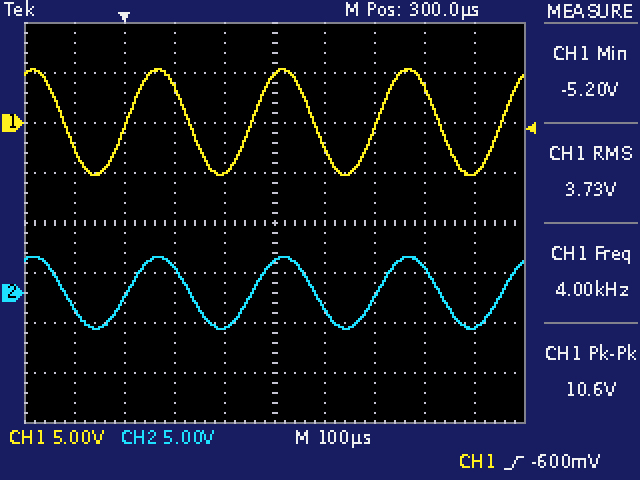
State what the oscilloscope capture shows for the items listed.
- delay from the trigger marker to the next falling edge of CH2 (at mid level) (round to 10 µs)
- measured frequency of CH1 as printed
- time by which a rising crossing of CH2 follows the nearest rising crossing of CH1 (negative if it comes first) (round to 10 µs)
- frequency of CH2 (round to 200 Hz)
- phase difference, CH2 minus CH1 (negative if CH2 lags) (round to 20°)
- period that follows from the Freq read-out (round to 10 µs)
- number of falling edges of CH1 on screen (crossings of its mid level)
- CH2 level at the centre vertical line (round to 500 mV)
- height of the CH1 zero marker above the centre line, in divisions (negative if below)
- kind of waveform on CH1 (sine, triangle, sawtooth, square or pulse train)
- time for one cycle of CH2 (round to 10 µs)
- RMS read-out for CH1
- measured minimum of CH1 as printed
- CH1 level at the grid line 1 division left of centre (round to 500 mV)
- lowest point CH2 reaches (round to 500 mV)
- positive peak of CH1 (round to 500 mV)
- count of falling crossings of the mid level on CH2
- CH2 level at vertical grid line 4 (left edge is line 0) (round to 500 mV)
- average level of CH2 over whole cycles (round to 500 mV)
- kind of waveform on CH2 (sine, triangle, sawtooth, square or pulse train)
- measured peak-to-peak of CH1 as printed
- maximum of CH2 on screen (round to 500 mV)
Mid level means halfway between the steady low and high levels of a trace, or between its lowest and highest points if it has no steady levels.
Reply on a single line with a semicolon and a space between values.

130 µs; 4.00 kHz; 0 µs; 4.0 kHz; 0°; 250 µs; 4; 3.0 V; +2.0 div; sine; 250 µs; 3.73 V; -5.20 V; -5.0 V; -3.5 V; 5.5 V; 4; -3.5 V; 0.0 V; sine; 10.6 V; 3.5 V
